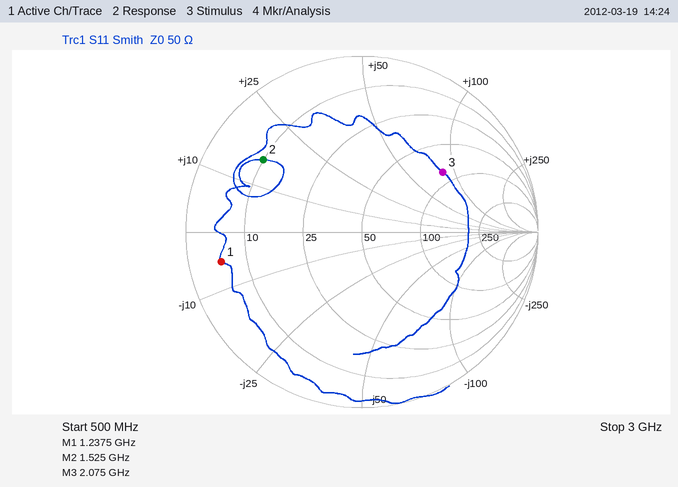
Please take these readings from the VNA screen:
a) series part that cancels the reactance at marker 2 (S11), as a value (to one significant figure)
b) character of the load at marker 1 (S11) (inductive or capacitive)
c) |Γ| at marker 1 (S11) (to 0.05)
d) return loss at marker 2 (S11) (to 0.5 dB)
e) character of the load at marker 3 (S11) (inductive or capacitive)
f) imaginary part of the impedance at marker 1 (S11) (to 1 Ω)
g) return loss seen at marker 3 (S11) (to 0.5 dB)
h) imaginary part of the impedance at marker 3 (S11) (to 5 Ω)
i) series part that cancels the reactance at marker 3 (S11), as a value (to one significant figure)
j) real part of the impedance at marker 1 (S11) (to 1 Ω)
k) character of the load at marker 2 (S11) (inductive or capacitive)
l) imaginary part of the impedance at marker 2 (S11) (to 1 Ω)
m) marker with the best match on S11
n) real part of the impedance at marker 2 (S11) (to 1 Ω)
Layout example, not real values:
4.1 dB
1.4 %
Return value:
7 pF
capacitive
0.80
3.0 dB
inductive
-5 Ω
5.0 dB
+85 Ω
900 fF
5 Ω
inductive
+16 Ω
marker 3
10 Ω
